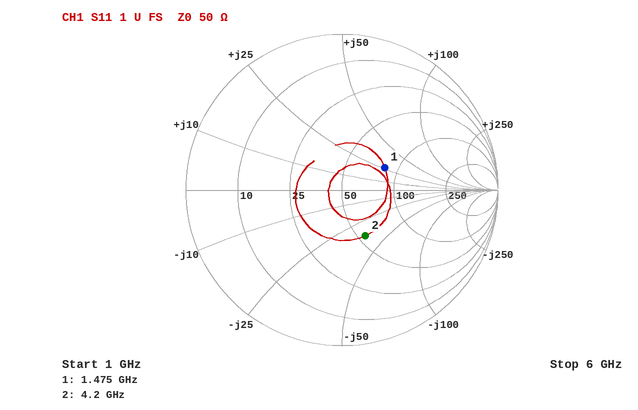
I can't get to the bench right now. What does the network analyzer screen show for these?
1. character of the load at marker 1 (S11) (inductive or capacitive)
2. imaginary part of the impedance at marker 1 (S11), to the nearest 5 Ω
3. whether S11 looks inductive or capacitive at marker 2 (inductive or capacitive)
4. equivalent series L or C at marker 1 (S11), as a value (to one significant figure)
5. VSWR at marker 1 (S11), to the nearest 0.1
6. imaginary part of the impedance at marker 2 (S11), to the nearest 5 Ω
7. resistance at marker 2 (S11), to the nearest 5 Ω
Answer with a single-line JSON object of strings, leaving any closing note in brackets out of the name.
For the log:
{"character of the load at marker 1 (S11)": "inductive", "imaginary part of the impedance at marker 1 (S11), to the nearest 5 Ω": "+25 Ω", "whether S11 looks inductive or capacitive at marker 2": "capacitive", "equivalent series L or C at marker 1 (S11), as a value": "3 nH", "VSWR at marker 1 (S11), to the nearest 0.1": "1.9", "imaginary part of the impedance at marker 2 (S11), to the nearest 5 Ω": "-35 Ω", "resistance at marker 2 (S11), to the nearest 5 Ω": "55 Ω"}
